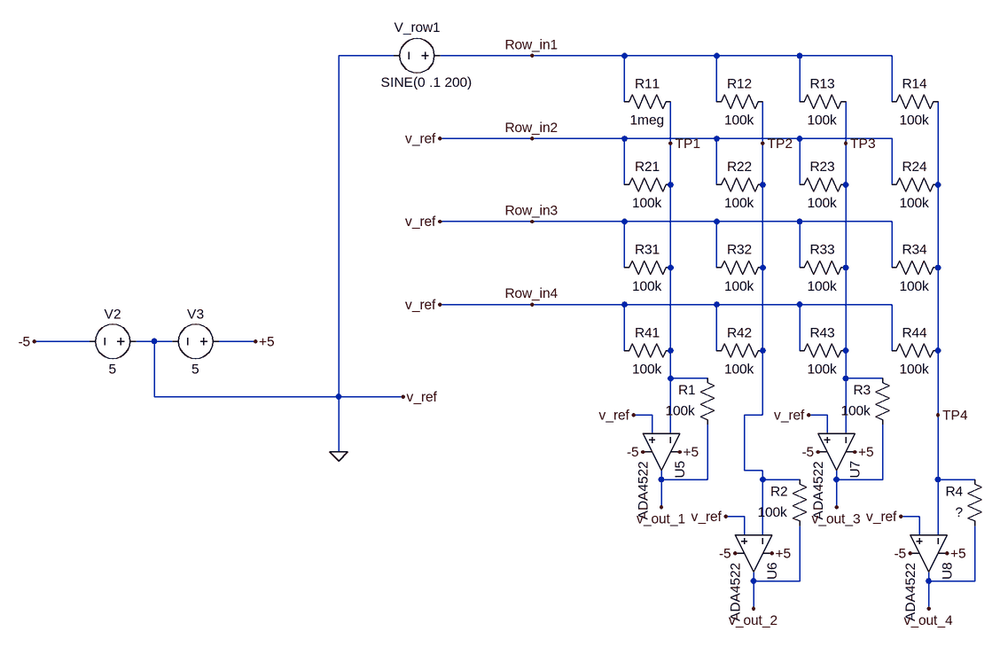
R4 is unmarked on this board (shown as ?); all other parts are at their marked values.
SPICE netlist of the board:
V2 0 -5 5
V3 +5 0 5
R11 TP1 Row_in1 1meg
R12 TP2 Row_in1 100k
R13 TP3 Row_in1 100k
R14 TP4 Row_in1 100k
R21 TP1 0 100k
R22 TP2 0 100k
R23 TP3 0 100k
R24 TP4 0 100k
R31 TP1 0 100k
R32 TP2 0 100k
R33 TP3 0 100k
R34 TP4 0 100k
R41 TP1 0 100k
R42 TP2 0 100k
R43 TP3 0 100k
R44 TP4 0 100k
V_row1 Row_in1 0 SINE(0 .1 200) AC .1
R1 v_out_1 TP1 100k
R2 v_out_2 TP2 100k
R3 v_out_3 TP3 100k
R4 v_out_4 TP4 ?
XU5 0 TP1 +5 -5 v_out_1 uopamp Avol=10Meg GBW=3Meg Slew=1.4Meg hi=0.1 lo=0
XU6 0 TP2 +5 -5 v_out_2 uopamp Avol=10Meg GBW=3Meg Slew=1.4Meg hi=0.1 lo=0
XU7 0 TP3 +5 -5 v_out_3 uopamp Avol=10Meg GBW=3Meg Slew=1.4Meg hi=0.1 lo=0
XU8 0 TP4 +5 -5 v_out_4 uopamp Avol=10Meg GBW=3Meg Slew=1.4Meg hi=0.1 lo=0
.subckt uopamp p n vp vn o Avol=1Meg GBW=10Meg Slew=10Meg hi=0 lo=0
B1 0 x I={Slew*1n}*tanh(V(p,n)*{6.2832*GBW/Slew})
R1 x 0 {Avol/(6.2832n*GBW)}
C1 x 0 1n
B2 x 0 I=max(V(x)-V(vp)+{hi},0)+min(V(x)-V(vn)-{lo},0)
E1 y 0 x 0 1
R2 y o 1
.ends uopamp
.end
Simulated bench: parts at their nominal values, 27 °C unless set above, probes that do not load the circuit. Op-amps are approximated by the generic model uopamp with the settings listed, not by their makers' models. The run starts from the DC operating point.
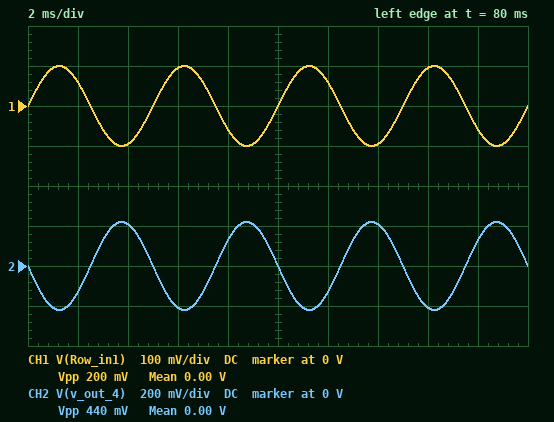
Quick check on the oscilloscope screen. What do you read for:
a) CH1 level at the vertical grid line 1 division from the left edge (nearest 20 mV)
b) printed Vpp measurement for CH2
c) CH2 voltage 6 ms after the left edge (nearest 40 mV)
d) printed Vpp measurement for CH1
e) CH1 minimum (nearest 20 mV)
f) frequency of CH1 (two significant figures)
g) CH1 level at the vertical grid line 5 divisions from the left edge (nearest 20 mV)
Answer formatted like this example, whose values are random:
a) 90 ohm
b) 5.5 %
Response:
a) 60 mV
b) 440 mV
c) -200 mV
d) 200 mV
e) -100 mV
f) 200 Hz
g) 0 V
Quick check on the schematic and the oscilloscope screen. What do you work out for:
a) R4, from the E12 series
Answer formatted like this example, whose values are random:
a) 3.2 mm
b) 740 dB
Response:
a) 220 kΩ
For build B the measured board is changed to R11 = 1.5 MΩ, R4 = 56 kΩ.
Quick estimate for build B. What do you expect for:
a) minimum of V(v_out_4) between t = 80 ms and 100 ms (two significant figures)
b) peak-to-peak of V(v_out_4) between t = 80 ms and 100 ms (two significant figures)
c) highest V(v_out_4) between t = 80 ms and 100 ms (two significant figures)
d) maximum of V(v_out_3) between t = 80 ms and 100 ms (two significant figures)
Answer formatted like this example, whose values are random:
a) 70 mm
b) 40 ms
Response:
a) -56 mV
b) 110 mV
c) 56 mV
d) 100 mV
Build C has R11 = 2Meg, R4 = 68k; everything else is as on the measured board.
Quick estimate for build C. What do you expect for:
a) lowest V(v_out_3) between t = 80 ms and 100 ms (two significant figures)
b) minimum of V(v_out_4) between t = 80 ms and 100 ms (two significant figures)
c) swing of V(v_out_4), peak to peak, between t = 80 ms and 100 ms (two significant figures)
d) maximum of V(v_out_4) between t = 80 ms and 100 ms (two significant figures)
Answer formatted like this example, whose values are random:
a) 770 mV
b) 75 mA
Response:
a) -100 mV
b) -68 mV
c) 140 mV
d) 68 mV
